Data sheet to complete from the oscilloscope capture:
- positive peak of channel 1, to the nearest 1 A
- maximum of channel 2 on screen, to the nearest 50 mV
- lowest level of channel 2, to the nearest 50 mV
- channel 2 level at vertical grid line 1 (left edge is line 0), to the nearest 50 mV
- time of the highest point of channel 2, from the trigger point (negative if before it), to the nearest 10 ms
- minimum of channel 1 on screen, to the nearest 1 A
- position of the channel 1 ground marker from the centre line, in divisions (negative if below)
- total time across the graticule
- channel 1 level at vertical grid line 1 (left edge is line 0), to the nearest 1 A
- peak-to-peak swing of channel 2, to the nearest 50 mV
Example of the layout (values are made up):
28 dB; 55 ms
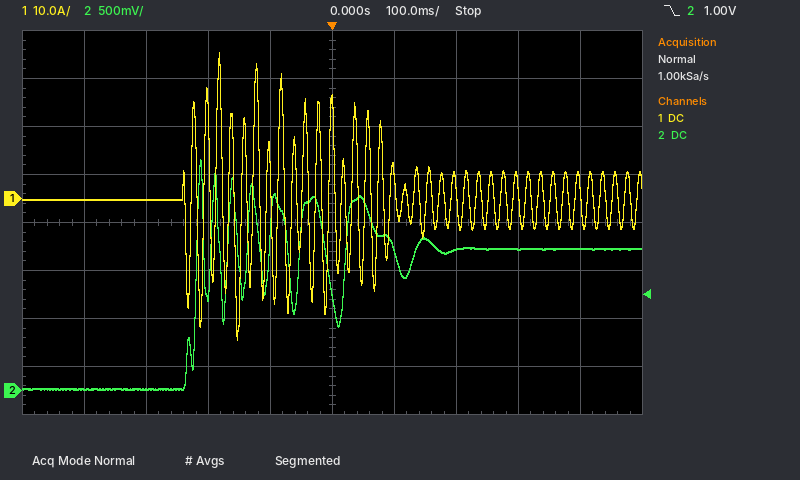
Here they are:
30 A; 2.40 V; 0 mV; 0 mV; -210 ms; -29 A; +0.5 div; 1 s; 0 A; 2.40 V
